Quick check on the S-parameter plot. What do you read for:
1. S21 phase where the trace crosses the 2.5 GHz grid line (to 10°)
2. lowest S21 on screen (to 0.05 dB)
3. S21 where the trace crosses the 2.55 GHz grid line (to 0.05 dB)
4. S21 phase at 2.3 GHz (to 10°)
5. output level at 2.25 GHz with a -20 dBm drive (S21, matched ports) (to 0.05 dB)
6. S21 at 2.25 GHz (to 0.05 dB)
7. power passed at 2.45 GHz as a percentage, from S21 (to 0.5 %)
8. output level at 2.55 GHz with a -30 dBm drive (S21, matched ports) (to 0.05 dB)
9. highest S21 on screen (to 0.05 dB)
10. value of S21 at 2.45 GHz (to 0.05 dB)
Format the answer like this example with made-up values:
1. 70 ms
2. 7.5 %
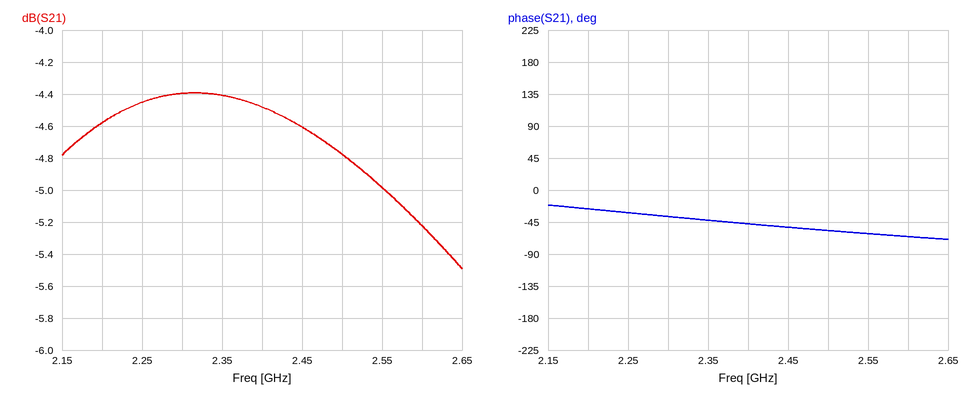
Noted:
1. -60°
2. -5.50 dB
3. -5.00 dB
4. -40°
5. -24.45 dBm
6. -4.45 dB
7. 34.5 %
8. -35.00 dBm
9. -4.40 dB
10. -4.60 dB
